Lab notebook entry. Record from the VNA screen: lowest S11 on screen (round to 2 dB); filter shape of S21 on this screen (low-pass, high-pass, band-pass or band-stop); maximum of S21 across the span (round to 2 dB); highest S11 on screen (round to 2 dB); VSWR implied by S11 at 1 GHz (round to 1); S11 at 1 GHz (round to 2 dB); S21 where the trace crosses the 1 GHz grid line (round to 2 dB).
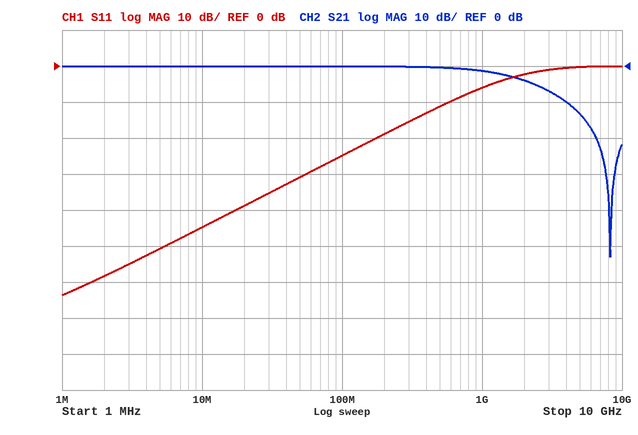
-64 dB
low-pass
0 dB
0 dB
3
-6 dB
-2 dB
